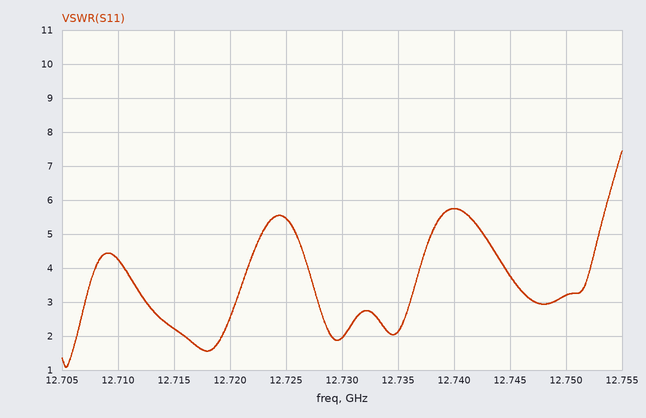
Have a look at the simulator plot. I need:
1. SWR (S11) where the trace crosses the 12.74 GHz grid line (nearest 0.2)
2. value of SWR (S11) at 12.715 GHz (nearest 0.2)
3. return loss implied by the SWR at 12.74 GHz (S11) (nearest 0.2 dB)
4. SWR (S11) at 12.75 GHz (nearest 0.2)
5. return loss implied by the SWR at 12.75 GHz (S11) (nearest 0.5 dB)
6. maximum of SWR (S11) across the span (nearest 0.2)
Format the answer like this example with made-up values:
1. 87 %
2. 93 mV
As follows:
1. 5.8
2. 2.2
3. 3.0 dB
4. 3.2
5. 5.5 dB
6. 7.4
